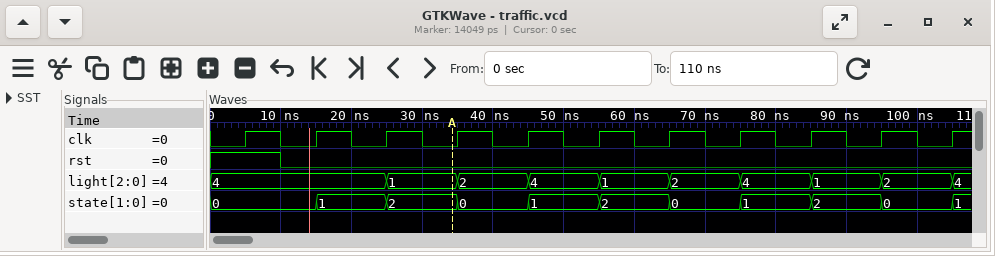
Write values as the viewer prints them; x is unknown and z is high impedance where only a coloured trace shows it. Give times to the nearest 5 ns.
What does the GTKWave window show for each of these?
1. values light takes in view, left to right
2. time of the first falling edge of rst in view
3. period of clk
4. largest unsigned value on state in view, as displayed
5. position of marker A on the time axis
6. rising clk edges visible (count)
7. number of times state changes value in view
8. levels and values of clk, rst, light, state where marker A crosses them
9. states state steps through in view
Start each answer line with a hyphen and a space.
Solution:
- 4, 1, 2, 4, 1, 2, 4, 1, 2, 4
- 10 ns
- 10 ns
- 2
- 35 ns
- 11
- 10
- clk=0, rst=0, light=1, state=2
- 0, 1, 2, 0, 1, 2, 0, 1, 2, 0, 1
